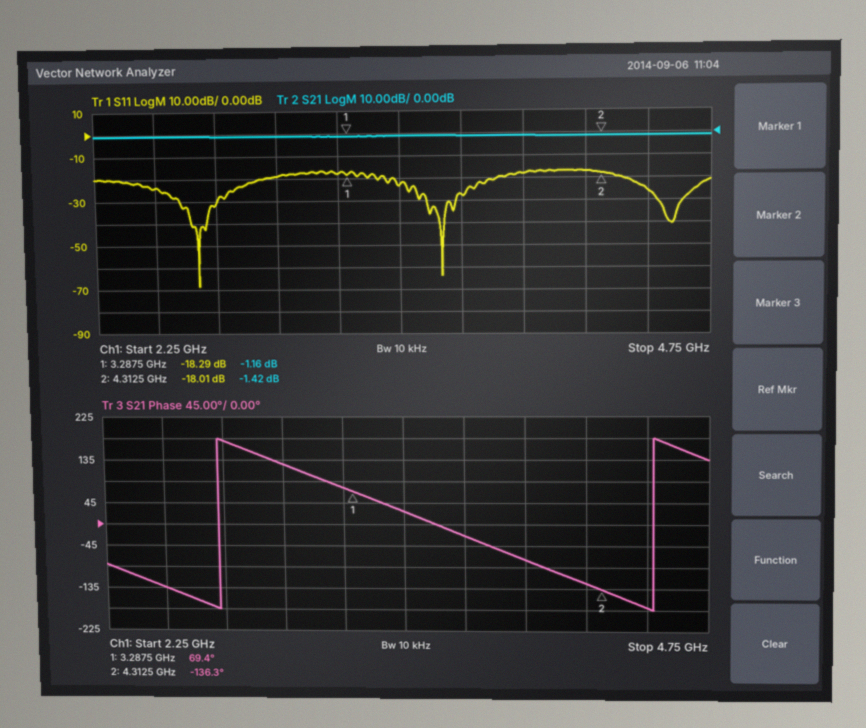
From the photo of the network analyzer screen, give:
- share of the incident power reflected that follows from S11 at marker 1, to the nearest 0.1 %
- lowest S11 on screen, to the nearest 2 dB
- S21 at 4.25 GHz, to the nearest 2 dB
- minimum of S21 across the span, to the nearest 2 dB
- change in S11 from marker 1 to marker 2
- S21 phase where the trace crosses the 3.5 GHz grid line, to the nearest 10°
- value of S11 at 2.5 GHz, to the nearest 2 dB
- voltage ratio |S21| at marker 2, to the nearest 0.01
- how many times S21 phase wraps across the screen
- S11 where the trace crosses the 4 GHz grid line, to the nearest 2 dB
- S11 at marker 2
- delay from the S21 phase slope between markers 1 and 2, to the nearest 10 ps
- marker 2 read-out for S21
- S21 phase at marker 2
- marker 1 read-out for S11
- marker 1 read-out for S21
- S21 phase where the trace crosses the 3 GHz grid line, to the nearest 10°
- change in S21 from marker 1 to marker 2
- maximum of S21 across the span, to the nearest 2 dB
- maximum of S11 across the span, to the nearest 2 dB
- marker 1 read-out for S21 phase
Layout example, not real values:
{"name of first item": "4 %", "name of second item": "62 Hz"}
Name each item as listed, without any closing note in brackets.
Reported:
{"share of the incident power reflected that follows from S11 at marker 1, to the nearest 0.1 %": "1.5 %", "lowest S11 on screen, to the nearest 2 dB": "-68 dB", "S21 at 4.25 GHz, to the nearest 2 dB": "-2 dB", "minimum of S21 across the span, to the nearest 2 dB": "-2 dB", "change in S11 from marker 1 to marker 2": "0.28 dB", "S21 phase where the trace crosses the 3.5 GHz grid line, to the nearest 10°": "30°", "value of S11 at 2.5 GHz, to the nearest 2 dB": "-24 dB", "voltage ratio |S21| at marker 2, to the nearest 0.01": "0.85", "how many times S21 phase wraps across the screen": "2", "S11 where the trace crosses the 4 GHz grid line, to the nearest 2 dB": "-18 dB", "S11 at marker 2": "-18.01 dB", "delay from the S21 phase slope between markers 1 and 2, to the nearest 10 ps": "560 ps", "marker 2 read-out for S21": "-1.42 dB", "S21 phase at marker 2": "-136.3°", "marker 1 read-out for S11": "-18.29 dB", "marker 1 read-out for S21": "-1.16 dB", "S21 phase where the trace crosses the 3 GHz grid line, to the nearest 10°": "130°", "change in S21 from marker 1 to marker 2": "-0.26 dB", "maximum of S21 across the span, to the nearest 2 dB": "0 dB", "maximum of S11 across the span, to the nearest 2 dB": "-16 dB", "marker 1 read-out for S21 phase": "69.4°"}
